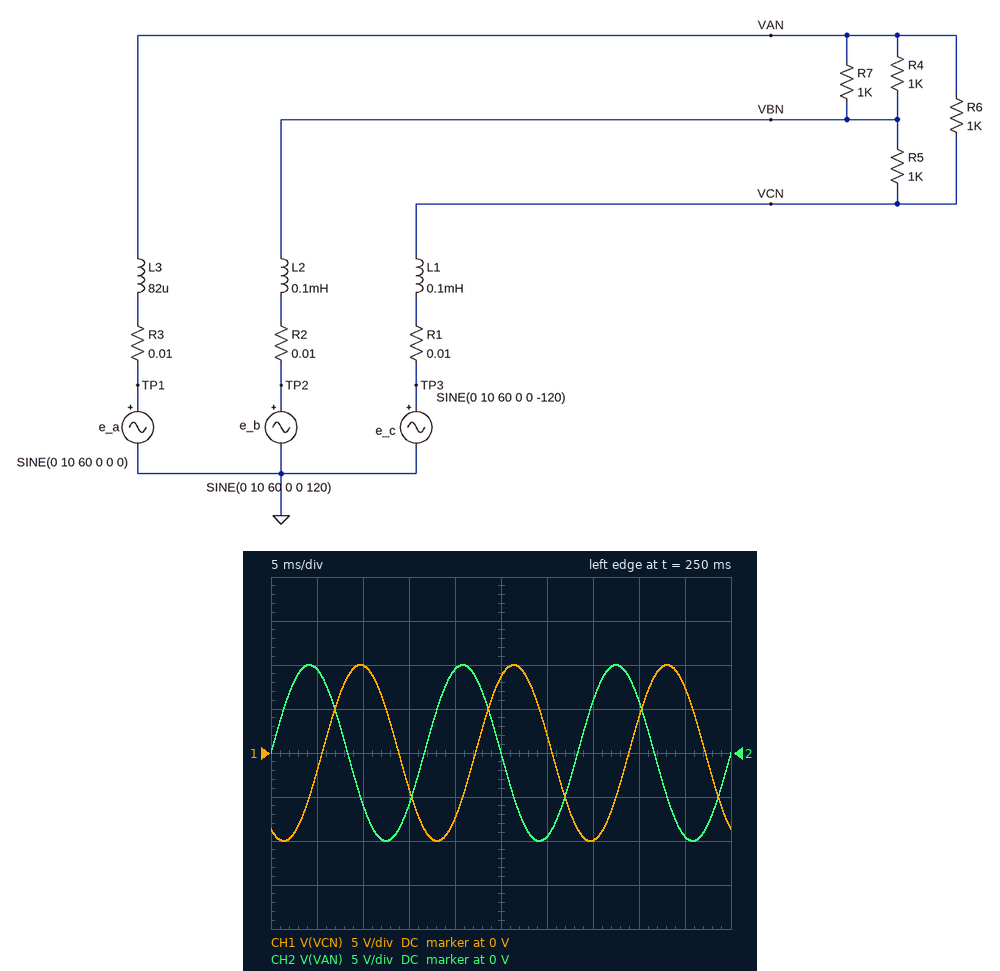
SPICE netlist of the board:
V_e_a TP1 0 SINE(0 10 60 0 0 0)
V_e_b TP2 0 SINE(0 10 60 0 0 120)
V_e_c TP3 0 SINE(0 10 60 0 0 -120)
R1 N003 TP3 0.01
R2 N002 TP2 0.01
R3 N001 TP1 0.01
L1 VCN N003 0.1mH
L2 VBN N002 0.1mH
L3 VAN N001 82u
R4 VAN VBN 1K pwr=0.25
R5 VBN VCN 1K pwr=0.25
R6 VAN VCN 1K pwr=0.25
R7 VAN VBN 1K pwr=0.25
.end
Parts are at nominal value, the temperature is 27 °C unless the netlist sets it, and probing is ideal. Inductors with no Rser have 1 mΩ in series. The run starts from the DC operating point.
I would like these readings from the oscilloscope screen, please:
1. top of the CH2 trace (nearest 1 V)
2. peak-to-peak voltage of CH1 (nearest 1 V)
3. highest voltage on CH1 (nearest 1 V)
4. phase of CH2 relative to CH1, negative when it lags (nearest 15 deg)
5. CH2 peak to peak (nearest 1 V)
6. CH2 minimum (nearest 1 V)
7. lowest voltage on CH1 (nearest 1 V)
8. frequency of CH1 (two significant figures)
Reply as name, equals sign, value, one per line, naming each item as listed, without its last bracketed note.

top of the CH2 trace = 10 V
peak-to-peak voltage of CH1 = 20 V
highest voltage on CH1 = 10 V
phase of CH2 relative to CH1, negative when it lags = 120 deg
CH2 peak to peak = 20 V
CH2 minimum = -10 V
lowest voltage on CH1 = -10 V
frequency of CH1 = 60 Hz
